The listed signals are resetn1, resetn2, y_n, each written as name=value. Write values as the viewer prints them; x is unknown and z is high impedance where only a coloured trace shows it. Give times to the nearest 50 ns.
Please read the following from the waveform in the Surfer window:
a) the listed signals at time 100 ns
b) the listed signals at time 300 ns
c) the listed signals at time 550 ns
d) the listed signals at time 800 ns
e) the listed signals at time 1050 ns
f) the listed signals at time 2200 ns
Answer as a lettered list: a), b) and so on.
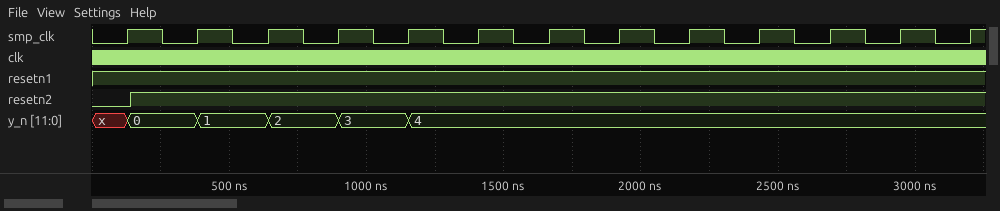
a) resetn1=1, resetn2=0, y_n=x
b) resetn1=1, resetn2=1, y_n=0
c) resetn1=1, resetn2=1, y_n=1
d) resetn1=1, resetn2=1, y_n=2
e) resetn1=1, resetn2=1, y_n=3
f) resetn1=1, resetn2=1, y_n=4
